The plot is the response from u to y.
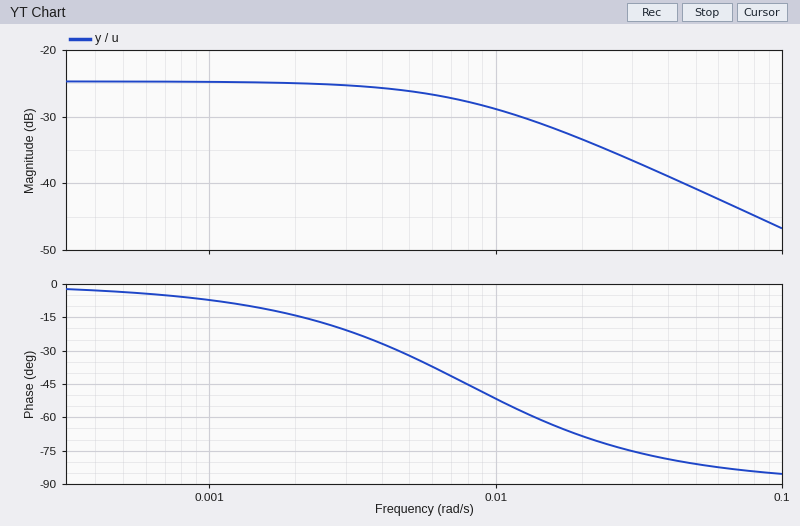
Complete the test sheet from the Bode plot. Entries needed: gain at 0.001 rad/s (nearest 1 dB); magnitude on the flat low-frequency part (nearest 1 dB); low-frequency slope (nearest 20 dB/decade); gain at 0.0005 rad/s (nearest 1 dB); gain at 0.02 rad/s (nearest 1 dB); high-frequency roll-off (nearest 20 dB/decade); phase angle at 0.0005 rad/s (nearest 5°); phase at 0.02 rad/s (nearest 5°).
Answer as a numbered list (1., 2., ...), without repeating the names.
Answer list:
1. -25 dB
2. -25 dB
3. 0 dB/decade
4. -25 dB
5. -33 dB
6. -20 dB/decade
7. -5°
8. -70°
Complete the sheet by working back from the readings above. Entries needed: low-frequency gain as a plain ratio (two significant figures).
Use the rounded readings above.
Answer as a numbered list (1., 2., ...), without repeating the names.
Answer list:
1. 0.056
